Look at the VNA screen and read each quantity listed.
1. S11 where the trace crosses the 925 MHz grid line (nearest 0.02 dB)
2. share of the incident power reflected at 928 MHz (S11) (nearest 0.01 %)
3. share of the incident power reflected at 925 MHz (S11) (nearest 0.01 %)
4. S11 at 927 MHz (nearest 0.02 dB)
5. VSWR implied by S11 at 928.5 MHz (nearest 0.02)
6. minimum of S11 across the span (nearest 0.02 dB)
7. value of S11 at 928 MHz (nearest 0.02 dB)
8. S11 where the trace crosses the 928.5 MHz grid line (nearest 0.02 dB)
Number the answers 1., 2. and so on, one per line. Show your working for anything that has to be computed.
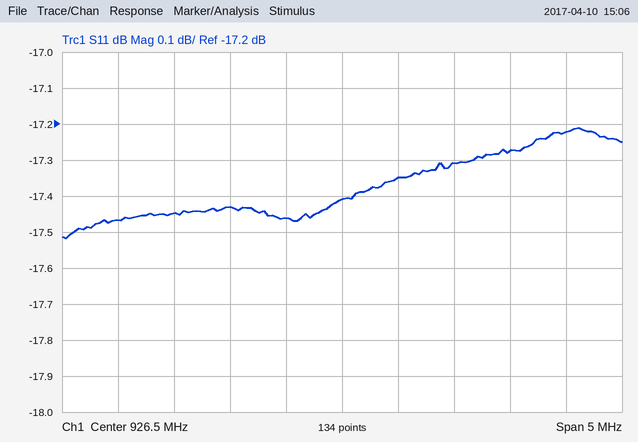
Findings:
1. -17.44 dB
2. 10^(-17.28/10) ≈ 1.87 %
3. 10^(-17.44/10) ≈ 1.80 %
4. -17.34 dB
5. |Γ| = 10^(-17.22/20) = 0.1377; VSWR = (1 + 0.1377)/(1 − 0.1377) ≈ 1.32
6. -17.52 dB
7. -17.28 dB
8. -17.22 dB
